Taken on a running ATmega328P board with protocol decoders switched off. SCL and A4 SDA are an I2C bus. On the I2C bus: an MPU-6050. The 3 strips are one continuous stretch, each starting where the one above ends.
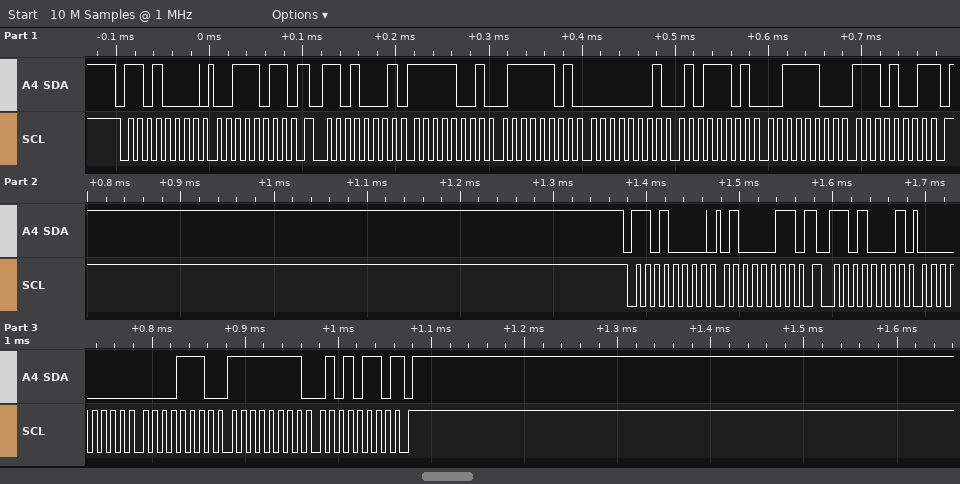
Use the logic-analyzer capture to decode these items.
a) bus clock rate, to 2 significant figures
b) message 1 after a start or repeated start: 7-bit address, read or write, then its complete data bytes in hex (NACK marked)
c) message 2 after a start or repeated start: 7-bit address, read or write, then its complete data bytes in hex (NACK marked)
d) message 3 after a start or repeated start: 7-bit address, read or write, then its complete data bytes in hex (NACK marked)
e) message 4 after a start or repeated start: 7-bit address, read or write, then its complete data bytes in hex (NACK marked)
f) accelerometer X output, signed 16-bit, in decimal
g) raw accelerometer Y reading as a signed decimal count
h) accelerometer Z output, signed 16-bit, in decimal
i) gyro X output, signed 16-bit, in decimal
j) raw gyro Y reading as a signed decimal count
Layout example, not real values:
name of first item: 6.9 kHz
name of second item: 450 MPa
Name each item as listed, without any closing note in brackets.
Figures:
bus clock rate, to 2 significant figures: 100 kHz
message 1 after a start or repeated start: 7-bit address, read or write, then its complete data bytes in hex: 0x68 write: 3B
message 2 after a start or repeated start: 7-bit address, read or write, then its complete data bytes in hex: 0x68 read: F9 7D 01 5D 3C E9 NACK
message 3 after a start or repeated start: 7-bit address, read or write, then its complete data bytes in hex: 0x68 write: 43
message 4 after a start or repeated start: 7-bit address, read or write, then its complete data bytes in hex: 0x68 read: 00 0E FF 56 NACK
accelerometer X output, signed 16-bit, in decimal: -1667
raw accelerometer Y reading as a signed decimal count: 349
accelerometer Z output, signed 16-bit, in decimal: 15593
gyro X output, signed 16-bit, in decimal: 14
raw gyro Y reading as a signed decimal count: -170
